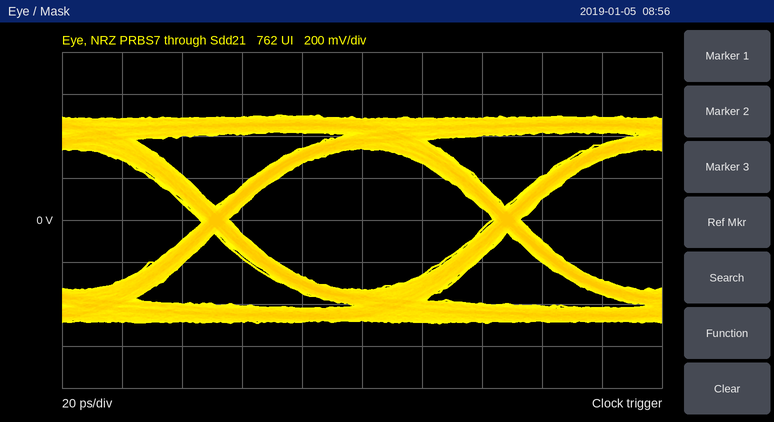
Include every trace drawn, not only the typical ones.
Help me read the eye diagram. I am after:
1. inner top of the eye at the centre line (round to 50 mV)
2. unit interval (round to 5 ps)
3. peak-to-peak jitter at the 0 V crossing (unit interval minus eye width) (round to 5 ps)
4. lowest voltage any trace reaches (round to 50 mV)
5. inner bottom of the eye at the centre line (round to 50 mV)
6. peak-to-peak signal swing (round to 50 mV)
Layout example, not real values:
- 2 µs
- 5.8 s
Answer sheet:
- 350 mV
- 95 ps
- 10 ps
- -500 mV
- -350 mV
- 1.00 V
